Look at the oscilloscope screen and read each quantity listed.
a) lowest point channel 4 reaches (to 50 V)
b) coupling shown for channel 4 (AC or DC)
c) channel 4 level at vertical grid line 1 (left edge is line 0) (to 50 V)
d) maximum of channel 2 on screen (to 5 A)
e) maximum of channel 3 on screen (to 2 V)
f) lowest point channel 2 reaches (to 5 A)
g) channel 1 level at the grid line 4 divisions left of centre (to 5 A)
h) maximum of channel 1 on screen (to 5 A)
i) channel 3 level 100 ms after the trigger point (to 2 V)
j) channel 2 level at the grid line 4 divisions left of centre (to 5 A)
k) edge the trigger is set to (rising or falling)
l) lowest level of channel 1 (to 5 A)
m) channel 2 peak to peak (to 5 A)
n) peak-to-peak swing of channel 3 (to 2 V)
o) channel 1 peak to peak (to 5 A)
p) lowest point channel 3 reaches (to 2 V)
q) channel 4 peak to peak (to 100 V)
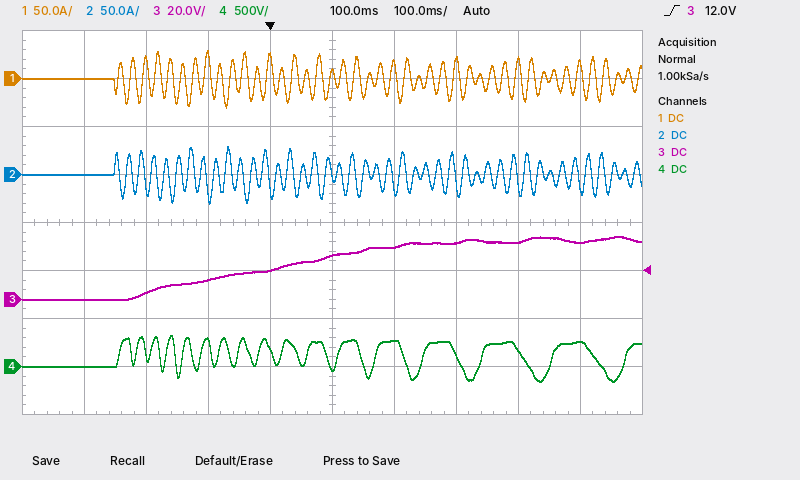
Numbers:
-150 V
DC
0 V
30 A
26 V
-30 A
0 A
30 A
18 V
0 A
rising
-30 A
60 A
26 V
60 A
0 V
500 V
